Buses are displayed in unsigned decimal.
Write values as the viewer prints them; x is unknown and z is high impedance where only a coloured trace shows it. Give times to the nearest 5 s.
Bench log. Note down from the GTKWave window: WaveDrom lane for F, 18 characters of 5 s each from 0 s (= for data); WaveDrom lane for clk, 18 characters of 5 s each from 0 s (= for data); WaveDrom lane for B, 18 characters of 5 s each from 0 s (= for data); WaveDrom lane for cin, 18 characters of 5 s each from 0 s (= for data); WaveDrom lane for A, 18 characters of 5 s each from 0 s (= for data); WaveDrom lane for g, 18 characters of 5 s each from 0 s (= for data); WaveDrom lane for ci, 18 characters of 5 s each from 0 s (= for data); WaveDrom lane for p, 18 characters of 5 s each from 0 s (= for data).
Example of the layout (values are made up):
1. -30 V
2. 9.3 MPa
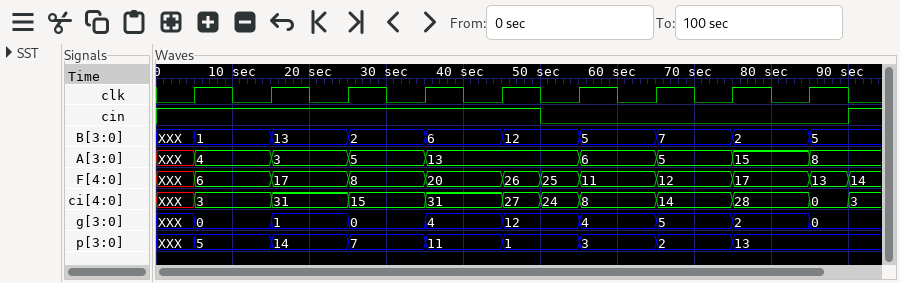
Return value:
1. {name: 'F', wave: 'x=.=.=.=.===.=.=.=', data: '6 17 8 20 26 25 11 12 17 13'}
2. {name: 'clk', wave: '010101010101010101'}
3. {name: 'B', wave: 'x=.=.=.=.=.=.=.=.=', data: '1 13 2 6 12 5 7 2 5'}
4. {name: 'cin', wave: '1.........0.......'}
5. {name: 'A', wave: 'x=.=.=.=...=.=.=.=', data: '4 3 5 13 6 5 15 8'}
6. {name: 'g', wave: 'x=.=.=.=.=.=.=.=.=', data: '0 1 0 4 12 4 5 2 0'}
7. {name: 'ci', wave: '==.=.=.=.===.=.=.=', data: 'XXX 3 31 15 31 27 24 8 14 28 0'}
8. {name: 'p', wave: 'x=.=.=.=.=.=.=.=..', data: '5 14 7 11 1 3 2 13'}
